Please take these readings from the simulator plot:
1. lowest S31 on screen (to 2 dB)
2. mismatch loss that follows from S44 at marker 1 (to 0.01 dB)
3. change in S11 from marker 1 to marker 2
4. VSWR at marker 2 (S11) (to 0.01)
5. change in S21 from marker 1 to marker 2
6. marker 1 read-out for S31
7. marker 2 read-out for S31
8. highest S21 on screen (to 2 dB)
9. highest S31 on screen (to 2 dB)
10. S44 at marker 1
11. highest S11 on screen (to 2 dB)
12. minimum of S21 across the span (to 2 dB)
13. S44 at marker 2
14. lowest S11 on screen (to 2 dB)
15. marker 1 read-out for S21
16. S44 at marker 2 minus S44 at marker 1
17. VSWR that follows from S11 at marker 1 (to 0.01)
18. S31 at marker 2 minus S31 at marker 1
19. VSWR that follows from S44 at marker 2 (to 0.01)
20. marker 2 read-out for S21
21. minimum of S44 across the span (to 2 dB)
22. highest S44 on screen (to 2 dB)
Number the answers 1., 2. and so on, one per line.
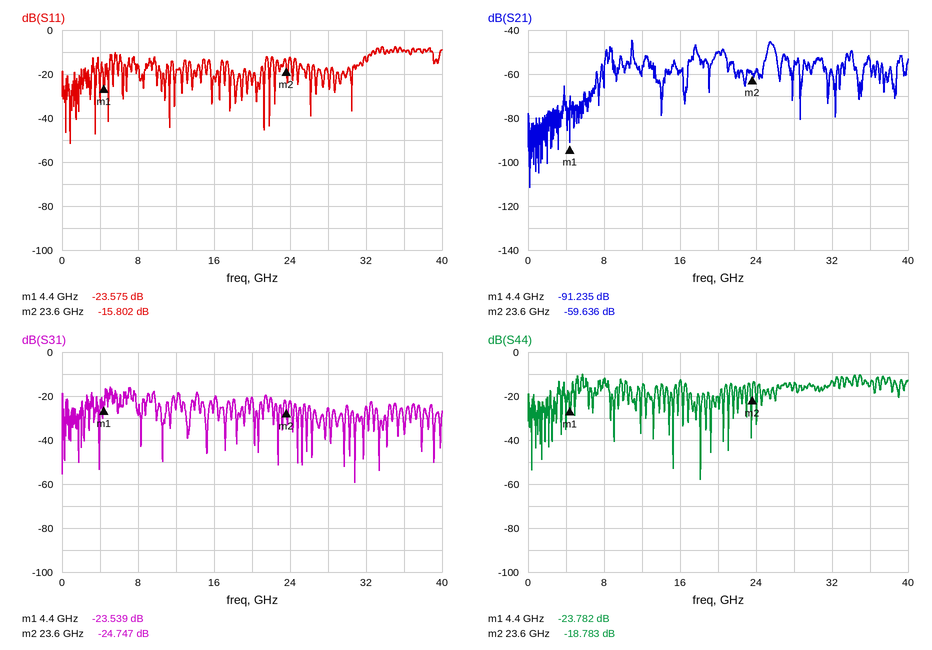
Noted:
1. -60 dB
2. 0.02 dB
3. 7.773 dB
4. 1.39
5. 31.599 dB
6. -23.539 dB
7. -24.747 dB
8. -44 dB
9. -16 dB
10. -23.782 dB
11. -8 dB
12. -112 dB
13. -18.783 dB
14. -52 dB
15. -91.235 dB
16. 4.999 dB
17. 1.14
18. -1.208 dB
19. 1.26
20. -59.636 dB
21. -58 dB
22. -10 dB
